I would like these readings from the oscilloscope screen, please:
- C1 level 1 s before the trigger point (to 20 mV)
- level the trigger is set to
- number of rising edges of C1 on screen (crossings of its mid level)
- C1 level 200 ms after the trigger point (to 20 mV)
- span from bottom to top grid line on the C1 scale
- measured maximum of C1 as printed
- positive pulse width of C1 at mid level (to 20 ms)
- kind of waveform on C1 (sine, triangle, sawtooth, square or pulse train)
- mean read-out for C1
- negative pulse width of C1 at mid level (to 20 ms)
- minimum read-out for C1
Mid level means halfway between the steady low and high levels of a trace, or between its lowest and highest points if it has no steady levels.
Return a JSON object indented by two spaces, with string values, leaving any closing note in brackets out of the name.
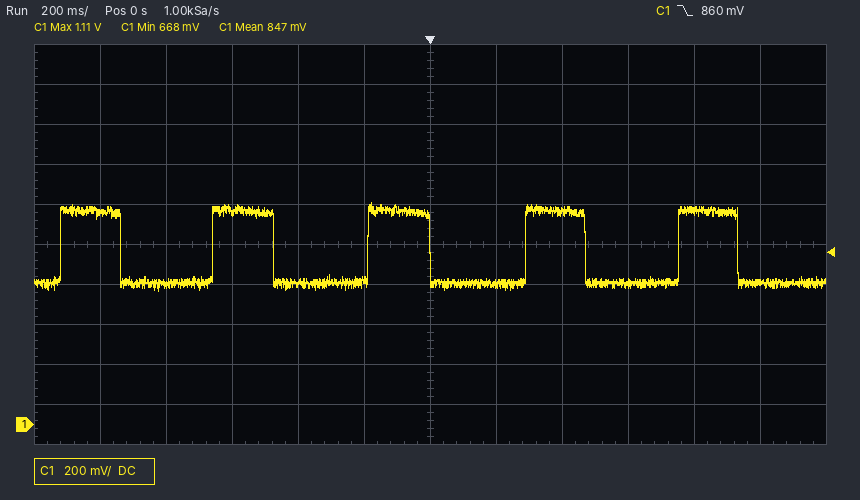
{
  "C1 level 1 s before the trigger point": "1.06 V",
  "level the trigger is set to": "860 mV",
  "number of rising edges of C1 on screen": "5",
  "C1 level 200 ms after the trigger point": "700 mV",
  "span from bottom to top grid line on the C1 scale": "2 V",
  "measured maximum of C1 as printed": "1.11 V",
  "positive pulse width of C1 at mid level": "180 ms",
  "kind of waveform on C1": "pulse train",
  "mean read-out for C1": "847 mV",
  "negative pulse width of C1 at mid level": "280 ms",
  "minimum read-out for C1": "668 mV"
}
